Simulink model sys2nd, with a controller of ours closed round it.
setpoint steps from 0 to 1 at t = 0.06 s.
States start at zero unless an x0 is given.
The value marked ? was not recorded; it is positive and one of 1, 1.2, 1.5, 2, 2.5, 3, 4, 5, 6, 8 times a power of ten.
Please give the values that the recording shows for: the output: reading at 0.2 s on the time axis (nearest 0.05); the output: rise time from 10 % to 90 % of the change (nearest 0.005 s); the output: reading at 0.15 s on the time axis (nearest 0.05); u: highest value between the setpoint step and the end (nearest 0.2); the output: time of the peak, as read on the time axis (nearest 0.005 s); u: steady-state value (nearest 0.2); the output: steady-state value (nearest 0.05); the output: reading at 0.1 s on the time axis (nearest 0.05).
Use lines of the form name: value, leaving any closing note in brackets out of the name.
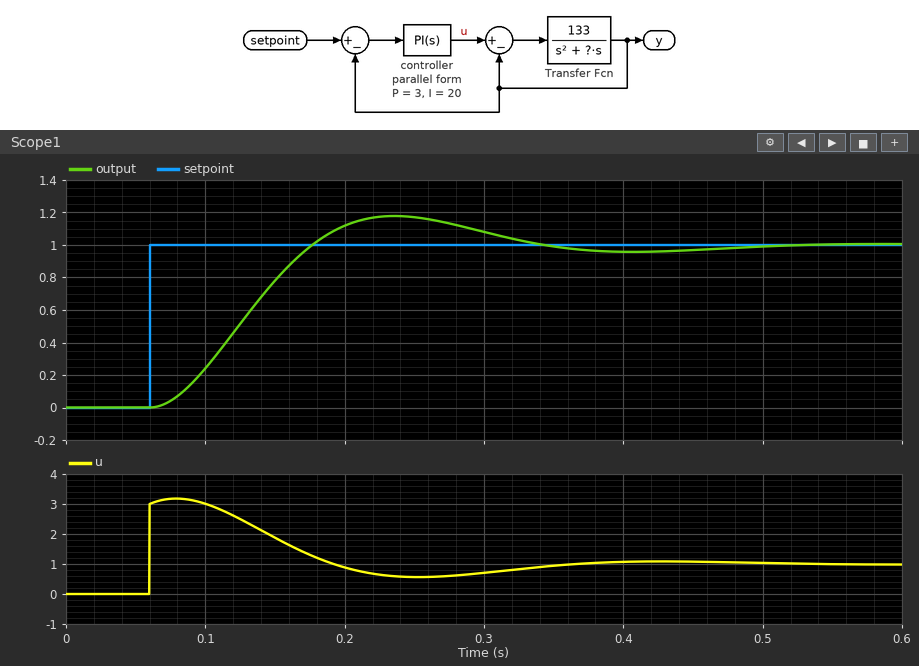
the output: reading at 0.2 s on the time axis: 1.10
the output: rise time from 10 % to 90 % of the change: 0.080 s
the output: reading at 0.15 s on the time axis: 0.80
u: highest value between the setpoint step and the end: 3.2
the output: time of the peak, as read on the time axis: 0.235 s
u: steady-state value: 1.0
the output: steady-state value: 1.00
the output: reading at 0.1 s on the time axis: 0.25
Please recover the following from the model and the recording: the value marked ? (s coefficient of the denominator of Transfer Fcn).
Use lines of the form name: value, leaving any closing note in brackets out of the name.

the value marked ?: 25
